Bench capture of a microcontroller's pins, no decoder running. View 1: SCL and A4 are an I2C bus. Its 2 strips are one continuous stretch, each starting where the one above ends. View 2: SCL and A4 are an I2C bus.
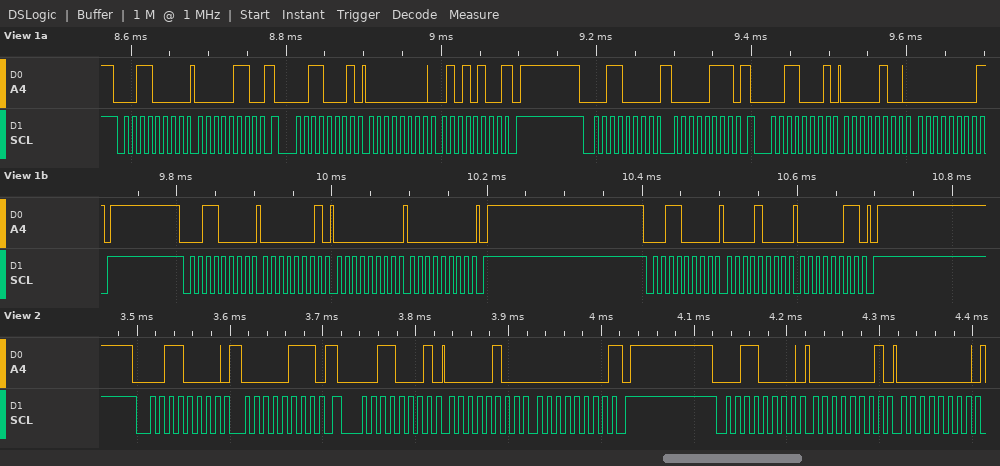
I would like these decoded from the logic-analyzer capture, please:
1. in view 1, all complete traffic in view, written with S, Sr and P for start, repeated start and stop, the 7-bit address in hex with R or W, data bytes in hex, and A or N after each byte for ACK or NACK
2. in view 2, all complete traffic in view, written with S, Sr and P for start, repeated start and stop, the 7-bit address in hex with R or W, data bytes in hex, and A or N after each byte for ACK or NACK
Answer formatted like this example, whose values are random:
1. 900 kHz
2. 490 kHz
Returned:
1. S 18W A 06 A Sr 18R A 00 A 54 N P S 18W A 07 A Sr 18R A 04 A 00 N P S 18W A 01 A 00 A 00 A P S 18W A 08 A 03 A P
2. S 18W A 07 A Sr 18R A 04 A 00 N P S 18W A 01 A 00 A
